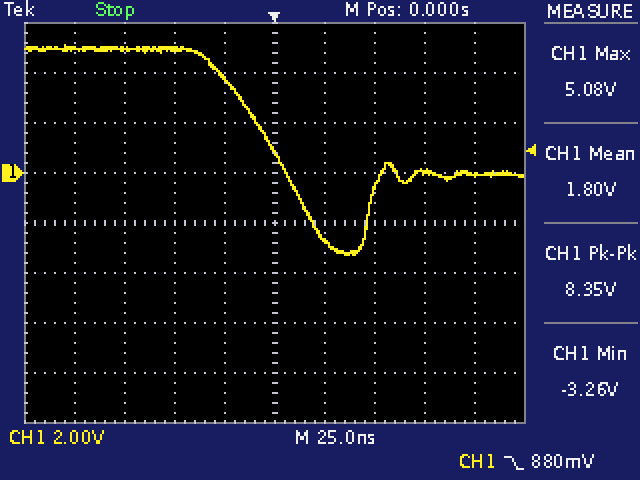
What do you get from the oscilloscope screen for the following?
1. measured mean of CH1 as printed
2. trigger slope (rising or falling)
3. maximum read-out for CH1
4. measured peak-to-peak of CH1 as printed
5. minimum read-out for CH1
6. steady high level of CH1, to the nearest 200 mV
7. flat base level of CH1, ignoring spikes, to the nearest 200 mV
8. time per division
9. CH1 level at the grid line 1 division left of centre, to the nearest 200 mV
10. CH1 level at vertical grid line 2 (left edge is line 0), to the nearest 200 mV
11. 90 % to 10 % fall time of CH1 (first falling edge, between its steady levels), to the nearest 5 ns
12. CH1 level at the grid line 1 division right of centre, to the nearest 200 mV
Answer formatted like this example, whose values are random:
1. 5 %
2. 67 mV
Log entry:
1. 1.80 V
2. falling
3. 5.08 V
4. 8.35 V
5. -3.26 V
6. 5.0 V
7. 0.0 V
8. 25 ns
9. 3.8 V
10. 5.0 V
11. 35 ns
12. -2.6 V
